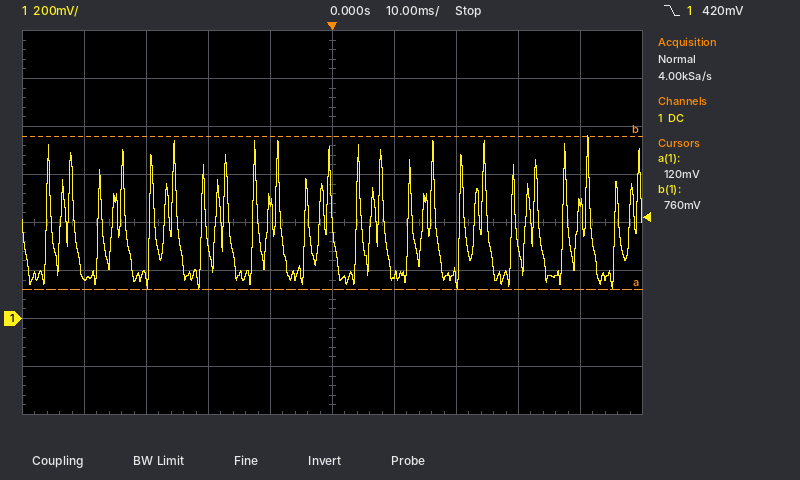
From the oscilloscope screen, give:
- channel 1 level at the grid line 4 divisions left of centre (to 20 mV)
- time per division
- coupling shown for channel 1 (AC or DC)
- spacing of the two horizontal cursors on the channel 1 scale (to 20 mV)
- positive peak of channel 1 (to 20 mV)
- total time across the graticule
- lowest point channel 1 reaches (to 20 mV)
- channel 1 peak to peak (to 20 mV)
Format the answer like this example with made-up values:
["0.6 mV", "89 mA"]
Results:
["180 mV", "10 ms", "DC", "640 mV", "760 mV", "100 ms", "120 mV", "640 mV"]
